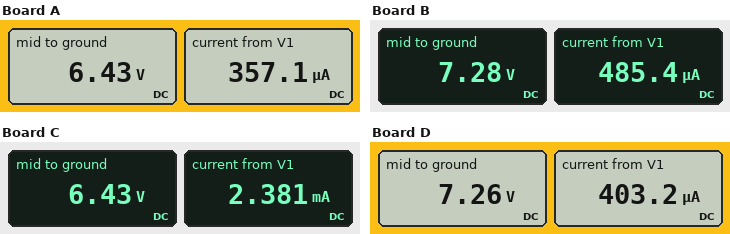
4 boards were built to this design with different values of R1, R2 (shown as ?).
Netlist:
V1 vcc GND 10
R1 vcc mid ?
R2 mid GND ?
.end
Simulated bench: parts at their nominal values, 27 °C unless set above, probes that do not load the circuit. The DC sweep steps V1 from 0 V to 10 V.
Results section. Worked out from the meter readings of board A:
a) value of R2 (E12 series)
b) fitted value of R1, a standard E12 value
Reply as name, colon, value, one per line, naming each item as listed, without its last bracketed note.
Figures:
value of R2: 18 kΩ
fitted value of R1, a standard E12 value: 10 kΩ
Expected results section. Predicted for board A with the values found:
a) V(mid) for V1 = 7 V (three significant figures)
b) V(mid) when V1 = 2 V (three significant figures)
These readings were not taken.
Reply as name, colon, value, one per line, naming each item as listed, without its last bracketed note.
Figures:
V(mid) for V1 = 7 V: 4.50 V
V(mid) when V1 = 2 V: 1.29 V
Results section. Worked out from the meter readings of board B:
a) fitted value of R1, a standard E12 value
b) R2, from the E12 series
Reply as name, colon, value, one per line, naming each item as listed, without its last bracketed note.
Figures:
fitted value of R1, a standard E12 value: 5.6 kΩ
R2, from the E12 series: 15 kΩ
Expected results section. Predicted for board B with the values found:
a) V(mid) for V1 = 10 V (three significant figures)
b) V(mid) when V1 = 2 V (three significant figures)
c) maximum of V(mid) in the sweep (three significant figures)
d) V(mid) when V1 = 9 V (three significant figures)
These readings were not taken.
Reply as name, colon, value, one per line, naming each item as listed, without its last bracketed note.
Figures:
V(mid) for V1 = 10 V: 7.28 V
V(mid) when V1 = 2 V: 1.46 V
maximum of V(mid) in the sweep: 7.28 V
V(mid) when V1 = 9 V: 6.55 V
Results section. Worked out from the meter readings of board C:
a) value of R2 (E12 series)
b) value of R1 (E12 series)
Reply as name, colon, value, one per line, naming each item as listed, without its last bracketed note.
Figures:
value of R2: 2.7 kΩ
value of R1: 1.5 kΩ
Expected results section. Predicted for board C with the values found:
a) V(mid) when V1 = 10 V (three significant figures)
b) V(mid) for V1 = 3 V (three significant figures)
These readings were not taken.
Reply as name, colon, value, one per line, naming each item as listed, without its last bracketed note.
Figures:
V(mid) when V1 = 10 V: 6.43 V
V(mid) for V1 = 3 V: 1.93 V
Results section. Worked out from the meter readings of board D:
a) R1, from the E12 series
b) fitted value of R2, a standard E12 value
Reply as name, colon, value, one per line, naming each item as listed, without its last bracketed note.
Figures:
R1, from the E12 series: 6.8 kΩ
fitted value of R2, a standard E12 value: 18 kΩ
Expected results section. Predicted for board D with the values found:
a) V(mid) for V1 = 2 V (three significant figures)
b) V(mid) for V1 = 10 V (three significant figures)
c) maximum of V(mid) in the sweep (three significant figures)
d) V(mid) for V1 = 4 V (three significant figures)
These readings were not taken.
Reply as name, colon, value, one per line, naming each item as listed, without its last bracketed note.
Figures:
V(mid) for V1 = 2 V: 1.45 V
V(mid) for V1 = 10 V: 7.26 V
maximum of V(mid) in the sweep: 7.26 V
V(mid) for V1 = 4 V: 2.90 V
